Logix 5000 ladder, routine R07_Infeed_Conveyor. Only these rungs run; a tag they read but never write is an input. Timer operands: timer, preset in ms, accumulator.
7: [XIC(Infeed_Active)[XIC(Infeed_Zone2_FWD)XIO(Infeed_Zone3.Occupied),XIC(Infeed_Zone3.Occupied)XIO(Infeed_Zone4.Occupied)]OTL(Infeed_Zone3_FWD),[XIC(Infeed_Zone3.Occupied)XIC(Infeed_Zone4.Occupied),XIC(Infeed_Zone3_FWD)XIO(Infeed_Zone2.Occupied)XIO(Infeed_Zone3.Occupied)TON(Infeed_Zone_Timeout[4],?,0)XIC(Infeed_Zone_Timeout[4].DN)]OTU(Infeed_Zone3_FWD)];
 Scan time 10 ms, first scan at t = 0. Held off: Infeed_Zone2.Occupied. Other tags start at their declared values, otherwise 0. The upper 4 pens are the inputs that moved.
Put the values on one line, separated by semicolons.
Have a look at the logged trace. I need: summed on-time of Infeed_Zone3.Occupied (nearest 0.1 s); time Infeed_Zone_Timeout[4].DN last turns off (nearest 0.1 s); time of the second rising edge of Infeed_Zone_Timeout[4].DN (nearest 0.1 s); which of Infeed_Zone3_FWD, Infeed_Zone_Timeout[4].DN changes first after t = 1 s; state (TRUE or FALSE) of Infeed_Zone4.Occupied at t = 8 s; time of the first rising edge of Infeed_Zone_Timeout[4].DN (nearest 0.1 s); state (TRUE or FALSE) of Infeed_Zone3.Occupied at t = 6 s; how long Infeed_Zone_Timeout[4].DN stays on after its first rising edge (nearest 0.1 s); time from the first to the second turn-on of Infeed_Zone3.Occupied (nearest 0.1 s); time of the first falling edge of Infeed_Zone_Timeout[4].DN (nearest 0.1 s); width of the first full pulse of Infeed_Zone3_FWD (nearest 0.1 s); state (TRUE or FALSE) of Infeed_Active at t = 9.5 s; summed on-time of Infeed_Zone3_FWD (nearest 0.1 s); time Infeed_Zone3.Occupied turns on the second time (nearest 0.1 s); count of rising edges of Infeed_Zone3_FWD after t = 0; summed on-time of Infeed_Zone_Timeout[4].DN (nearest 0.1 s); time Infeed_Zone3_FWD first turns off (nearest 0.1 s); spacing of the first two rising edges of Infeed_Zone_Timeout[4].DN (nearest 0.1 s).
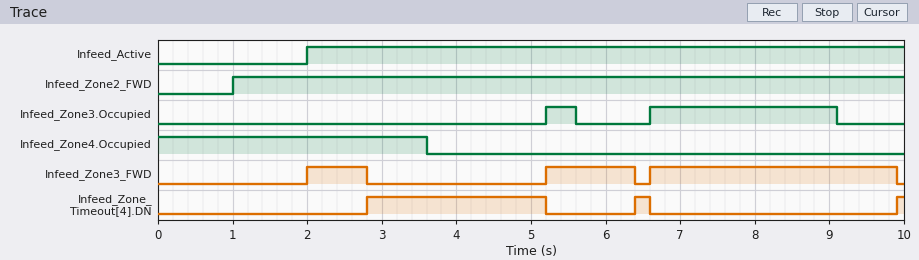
2.9 s; 6.6 s; 6.4 s; Infeed_Zone3_FWD; FALSE; 2.8 s; FALSE; 2.4 s; 1.4 s; 5.2 s; 0.8 s; TRUE; 5.3 s; 6.6 s; 3; 2.7 s; 2.8 s; 3.6 s
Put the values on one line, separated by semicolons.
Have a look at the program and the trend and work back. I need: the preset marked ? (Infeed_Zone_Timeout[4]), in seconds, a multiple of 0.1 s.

0.8 s
